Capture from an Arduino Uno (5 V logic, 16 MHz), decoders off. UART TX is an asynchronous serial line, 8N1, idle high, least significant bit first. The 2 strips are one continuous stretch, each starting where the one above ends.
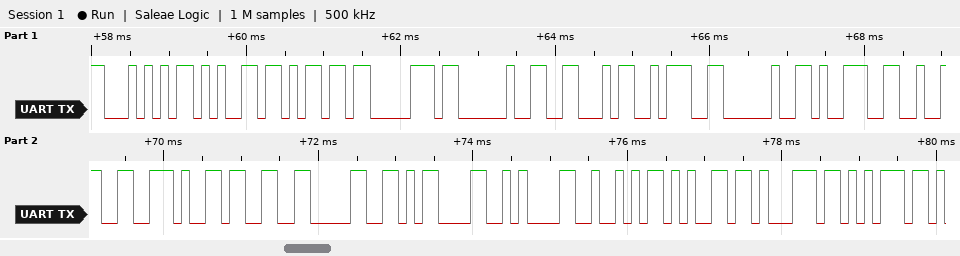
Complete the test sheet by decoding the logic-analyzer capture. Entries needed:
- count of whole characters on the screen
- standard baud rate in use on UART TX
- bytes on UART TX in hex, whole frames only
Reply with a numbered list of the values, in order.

1. 19
2. 9600 baud
3. 54 65 6D 70 20 46 3A 20 39 32 2E 33 30 0D 0A 52 65 71 75
